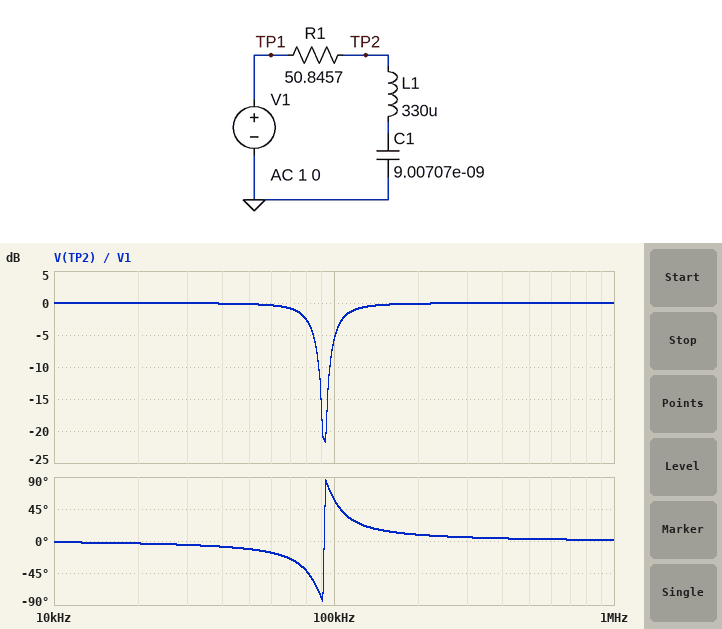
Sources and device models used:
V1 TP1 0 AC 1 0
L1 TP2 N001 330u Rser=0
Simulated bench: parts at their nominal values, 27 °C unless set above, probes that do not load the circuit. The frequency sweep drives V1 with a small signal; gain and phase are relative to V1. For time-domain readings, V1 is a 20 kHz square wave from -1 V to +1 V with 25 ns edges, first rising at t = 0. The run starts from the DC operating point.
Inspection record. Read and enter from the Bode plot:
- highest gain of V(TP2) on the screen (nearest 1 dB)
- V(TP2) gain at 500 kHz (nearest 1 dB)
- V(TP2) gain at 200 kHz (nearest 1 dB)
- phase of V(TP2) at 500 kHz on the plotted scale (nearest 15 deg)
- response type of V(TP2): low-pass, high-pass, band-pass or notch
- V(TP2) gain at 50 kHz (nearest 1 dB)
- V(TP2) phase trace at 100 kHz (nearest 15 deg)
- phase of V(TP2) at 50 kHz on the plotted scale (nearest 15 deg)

0 dB
0 dB
0 dB
0 deg
notch
0 dB
60 deg
-15 deg
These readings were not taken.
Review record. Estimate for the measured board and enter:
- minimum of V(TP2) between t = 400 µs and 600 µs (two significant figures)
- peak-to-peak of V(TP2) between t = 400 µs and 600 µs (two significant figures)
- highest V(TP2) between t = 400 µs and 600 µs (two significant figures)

-1.3 V
2.6 V
1.3 V
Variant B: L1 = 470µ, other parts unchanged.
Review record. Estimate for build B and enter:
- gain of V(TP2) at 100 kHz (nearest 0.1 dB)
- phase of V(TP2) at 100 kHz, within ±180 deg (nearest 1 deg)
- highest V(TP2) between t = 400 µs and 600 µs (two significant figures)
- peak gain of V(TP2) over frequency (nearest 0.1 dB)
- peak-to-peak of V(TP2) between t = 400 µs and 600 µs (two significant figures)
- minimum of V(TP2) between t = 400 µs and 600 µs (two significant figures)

-0.7 dB
23 deg
1.2 V
0 dB
2.4 V
-1.2 V
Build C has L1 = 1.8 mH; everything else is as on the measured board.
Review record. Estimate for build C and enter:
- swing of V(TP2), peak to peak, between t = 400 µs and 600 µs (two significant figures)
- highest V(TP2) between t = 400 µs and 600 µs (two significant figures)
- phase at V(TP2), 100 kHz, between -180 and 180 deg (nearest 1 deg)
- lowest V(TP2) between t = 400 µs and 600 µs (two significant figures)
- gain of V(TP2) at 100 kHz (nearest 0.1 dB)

2.2 V
1.1 V
3 deg
-1.1 V
0 dB
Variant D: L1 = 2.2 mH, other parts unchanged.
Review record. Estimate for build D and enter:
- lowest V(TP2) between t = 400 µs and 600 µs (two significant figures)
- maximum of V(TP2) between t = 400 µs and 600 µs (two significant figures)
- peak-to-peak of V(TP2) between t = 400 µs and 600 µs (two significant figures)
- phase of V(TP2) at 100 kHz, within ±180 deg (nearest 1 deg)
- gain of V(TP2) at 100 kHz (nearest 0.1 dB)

-1.1 V
1.1 V
2.2 V
2 deg
0 dB
